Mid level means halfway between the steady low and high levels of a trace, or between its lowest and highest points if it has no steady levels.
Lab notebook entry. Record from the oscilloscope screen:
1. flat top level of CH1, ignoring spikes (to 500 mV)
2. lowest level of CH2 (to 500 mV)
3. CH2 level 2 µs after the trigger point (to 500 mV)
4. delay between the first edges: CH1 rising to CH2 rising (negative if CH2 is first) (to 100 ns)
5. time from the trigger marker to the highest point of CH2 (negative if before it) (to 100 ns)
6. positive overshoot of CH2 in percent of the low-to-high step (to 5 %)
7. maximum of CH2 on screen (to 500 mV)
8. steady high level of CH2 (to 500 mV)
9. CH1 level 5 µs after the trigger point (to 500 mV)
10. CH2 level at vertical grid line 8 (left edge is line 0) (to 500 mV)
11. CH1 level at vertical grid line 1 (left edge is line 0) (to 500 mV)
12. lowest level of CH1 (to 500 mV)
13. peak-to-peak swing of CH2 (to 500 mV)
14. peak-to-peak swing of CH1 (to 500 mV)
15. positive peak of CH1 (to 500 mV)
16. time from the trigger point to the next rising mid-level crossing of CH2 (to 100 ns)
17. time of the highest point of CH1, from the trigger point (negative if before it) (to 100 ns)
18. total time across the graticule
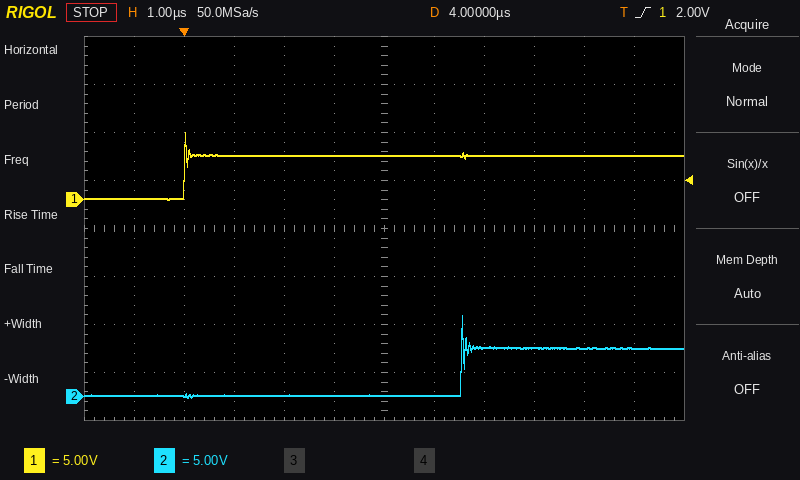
4.5 V
0.0 V
0.0 V
+5.5 µs
+5.6 µs
70 %
8.5 V
5.0 V
4.5 V
5.0 V
0.0 V
0.0 V
8.5 V
7.0 V
7.0 V
5.5 µs
0.0 µs
12 µs
